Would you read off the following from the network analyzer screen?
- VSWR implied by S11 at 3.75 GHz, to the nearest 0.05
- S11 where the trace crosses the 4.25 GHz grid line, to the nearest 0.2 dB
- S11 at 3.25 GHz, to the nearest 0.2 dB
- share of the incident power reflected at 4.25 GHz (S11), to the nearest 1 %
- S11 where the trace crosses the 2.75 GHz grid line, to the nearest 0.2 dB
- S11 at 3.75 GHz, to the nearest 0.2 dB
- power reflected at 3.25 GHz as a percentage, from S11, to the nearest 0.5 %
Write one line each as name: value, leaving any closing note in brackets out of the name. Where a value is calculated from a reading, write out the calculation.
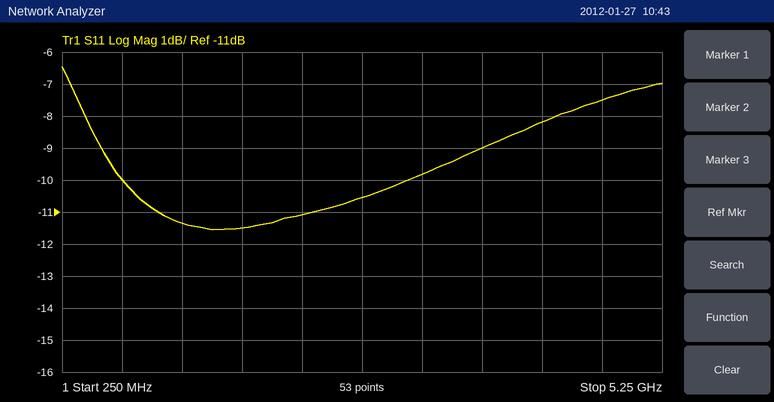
VSWR implied by S11 at 3.75 GHz, to the nearest 0.05: |Γ| = 10^(-9/20) = 0.3548; VSWR = (1 + 0.3548)/(1 − 0.3548) ≈ 2.10
S11 where the trace crosses the 4.25 GHz grid line, to the nearest 0.2 dB: -8.2 dB
S11 at 3.25 GHz, to the nearest 0.2 dB: -9.8 dB
share of the incident power reflected at 4.25 GHz (S11), to the nearest 1 %: 10^(-8.2/10) ≈ 15 %
S11 where the trace crosses the 2.75 GHz grid line, to the nearest 0.2 dB: -10.6 dB
S11 at 3.75 GHz, to the nearest 0.2 dB: -9.0 dB
power reflected at 3.25 GHz as a percentage, from S11, to the nearest 0.5 %: 10^(-9.8/10) ≈ 10.5 %
